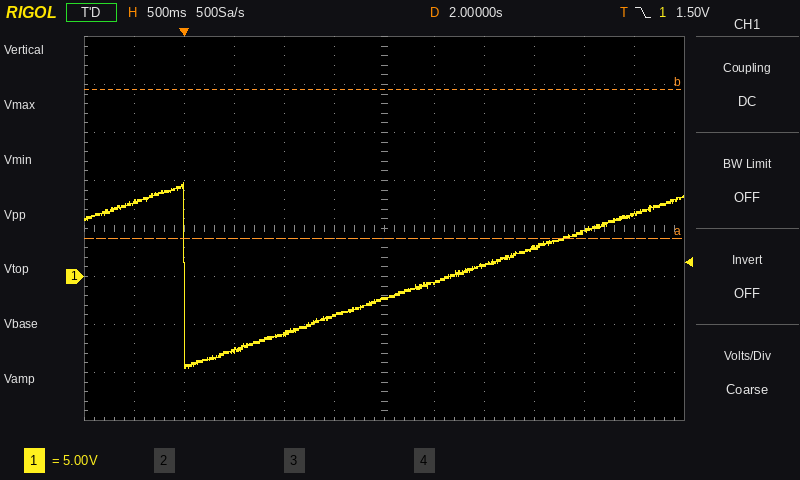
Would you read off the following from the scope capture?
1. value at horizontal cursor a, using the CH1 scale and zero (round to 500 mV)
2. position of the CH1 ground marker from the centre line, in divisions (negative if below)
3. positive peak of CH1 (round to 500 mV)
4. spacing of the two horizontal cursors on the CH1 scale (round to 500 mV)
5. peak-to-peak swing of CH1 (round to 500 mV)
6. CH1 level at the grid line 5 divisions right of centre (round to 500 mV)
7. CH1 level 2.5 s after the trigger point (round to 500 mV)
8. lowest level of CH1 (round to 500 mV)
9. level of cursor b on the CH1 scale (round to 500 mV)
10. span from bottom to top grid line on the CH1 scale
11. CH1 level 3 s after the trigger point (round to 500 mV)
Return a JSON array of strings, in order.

["4.0 V", "-1.0 div", "10.0 V", "15.5 V", "19.5 V", "6.5 V", "-500 mV", "-9.5 V", "19.5 V", "40 V", "1.0 V"]
